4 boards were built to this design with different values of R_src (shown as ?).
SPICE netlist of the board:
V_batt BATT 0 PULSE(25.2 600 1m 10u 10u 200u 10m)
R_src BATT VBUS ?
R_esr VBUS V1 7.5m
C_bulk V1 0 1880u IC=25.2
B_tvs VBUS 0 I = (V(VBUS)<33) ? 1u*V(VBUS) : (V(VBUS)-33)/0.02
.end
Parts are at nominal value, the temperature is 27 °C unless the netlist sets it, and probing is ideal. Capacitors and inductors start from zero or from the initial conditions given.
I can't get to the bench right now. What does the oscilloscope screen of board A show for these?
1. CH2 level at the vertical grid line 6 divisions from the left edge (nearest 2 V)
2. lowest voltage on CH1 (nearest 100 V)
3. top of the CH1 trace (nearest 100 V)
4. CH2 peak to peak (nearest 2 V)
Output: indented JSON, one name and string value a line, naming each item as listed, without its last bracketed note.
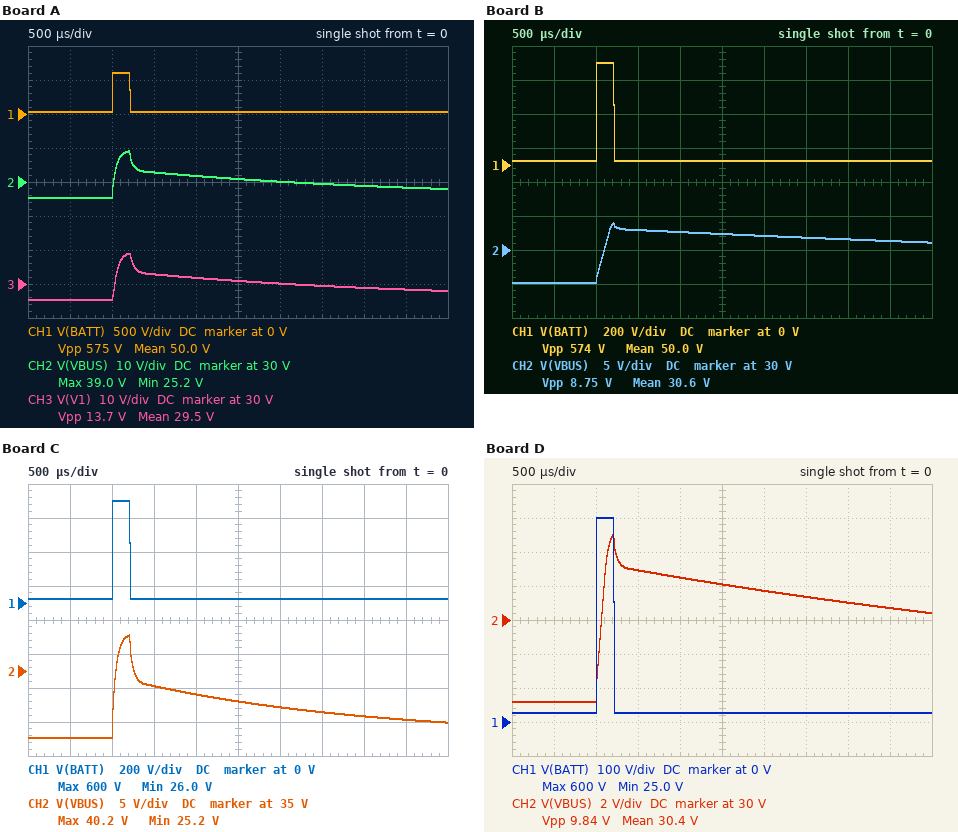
{
  "CH2 level at the vertical grid line 6 divisions from the left edge": "30 V",
  "lowest voltage on CH1": "0 V",
  "top of the CH1 trace": "600 V",
  "CH2 peak to peak": "14 V"
}
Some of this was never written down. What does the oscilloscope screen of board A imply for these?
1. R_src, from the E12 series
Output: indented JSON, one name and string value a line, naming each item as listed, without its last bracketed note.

{
  "R_src, from the E12 series": "1.8 Ω"
}
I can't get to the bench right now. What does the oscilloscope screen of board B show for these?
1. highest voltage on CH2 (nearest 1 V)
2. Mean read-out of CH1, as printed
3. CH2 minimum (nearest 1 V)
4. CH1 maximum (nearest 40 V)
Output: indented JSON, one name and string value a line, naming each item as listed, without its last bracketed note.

{
  "highest voltage on CH2": "34 V",
  "Mean read-out of CH1, as printed": "50.0 V",
  "CH2 minimum": "25 V",
  "CH1 maximum": "600 V"
}
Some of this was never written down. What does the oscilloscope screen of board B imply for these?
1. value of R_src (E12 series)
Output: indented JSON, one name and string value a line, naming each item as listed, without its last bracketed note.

{
  "value of R_src": "6.8 Ω"
}
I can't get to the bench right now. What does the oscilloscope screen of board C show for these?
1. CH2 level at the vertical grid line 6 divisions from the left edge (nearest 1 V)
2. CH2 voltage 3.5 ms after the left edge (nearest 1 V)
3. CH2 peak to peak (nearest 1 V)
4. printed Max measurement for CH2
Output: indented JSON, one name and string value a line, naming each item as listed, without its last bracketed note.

{
  "CH2 level at the vertical grid line 6 divisions from the left edge": "30 V",
  "CH2 voltage 3.5 ms after the left edge": "29 V",
  "CH2 peak to peak": "15 V",
  "printed Max measurement for CH2": "40.2 V"
}
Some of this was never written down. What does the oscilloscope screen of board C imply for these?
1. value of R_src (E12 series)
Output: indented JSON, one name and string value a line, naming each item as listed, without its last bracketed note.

{
  "value of R_src": "1.5 Ω"
}
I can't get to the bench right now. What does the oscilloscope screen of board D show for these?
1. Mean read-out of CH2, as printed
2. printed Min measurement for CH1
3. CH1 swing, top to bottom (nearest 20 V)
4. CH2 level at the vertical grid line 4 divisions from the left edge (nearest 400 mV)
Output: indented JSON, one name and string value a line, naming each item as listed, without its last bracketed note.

{
  "Mean read-out of CH2, as printed": "30.4 V",
  "printed Min measurement for CH1": "25.0 V",
  "CH1 swing, top to bottom": "580 V",
  "CH2 level at the vertical grid line 4 divisions from the left edge": "32.4 V"
}
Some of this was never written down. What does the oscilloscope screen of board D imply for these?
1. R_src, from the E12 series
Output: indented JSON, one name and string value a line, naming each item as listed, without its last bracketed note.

{
  "R_src, from the E12 series": "4.7 Ω"
}
